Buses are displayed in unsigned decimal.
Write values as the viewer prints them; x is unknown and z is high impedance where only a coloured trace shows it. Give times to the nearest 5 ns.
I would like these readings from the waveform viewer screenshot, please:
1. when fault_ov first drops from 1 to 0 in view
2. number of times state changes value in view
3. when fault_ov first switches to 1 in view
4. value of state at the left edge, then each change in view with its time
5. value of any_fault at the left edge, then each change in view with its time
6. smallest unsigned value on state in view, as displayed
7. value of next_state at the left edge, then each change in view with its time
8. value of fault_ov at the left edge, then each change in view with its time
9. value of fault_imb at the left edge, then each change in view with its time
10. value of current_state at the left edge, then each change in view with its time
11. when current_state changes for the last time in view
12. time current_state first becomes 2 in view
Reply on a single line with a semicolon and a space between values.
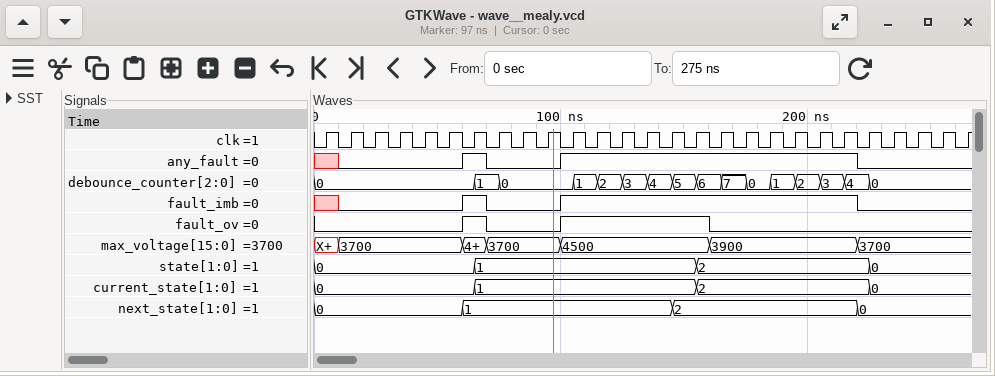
70 ns; 3; 60 ns; 0, 1 at 65 ns, 2 at 155 ns, 0 at 225 ns; x, 0 at 10 ns, 1 at 60 ns, 0 at 70 ns, 1 at 100 ns, 0 at 220 ns; 0; 0, 1 at 60 ns, 2 at 145 ns, 0 at 220 ns; 0, 1 at 60 ns, 0 at 70 ns, 1 at 100 ns, 0 at 160 ns; x, 0 at 10 ns, 1 at 60 ns, 0 at 70 ns, 1 at 100 ns, 0 at 220 ns; 0, 1 at 65 ns, 2 at 155 ns, 0 at 225 ns; 225 ns; 155 ns
